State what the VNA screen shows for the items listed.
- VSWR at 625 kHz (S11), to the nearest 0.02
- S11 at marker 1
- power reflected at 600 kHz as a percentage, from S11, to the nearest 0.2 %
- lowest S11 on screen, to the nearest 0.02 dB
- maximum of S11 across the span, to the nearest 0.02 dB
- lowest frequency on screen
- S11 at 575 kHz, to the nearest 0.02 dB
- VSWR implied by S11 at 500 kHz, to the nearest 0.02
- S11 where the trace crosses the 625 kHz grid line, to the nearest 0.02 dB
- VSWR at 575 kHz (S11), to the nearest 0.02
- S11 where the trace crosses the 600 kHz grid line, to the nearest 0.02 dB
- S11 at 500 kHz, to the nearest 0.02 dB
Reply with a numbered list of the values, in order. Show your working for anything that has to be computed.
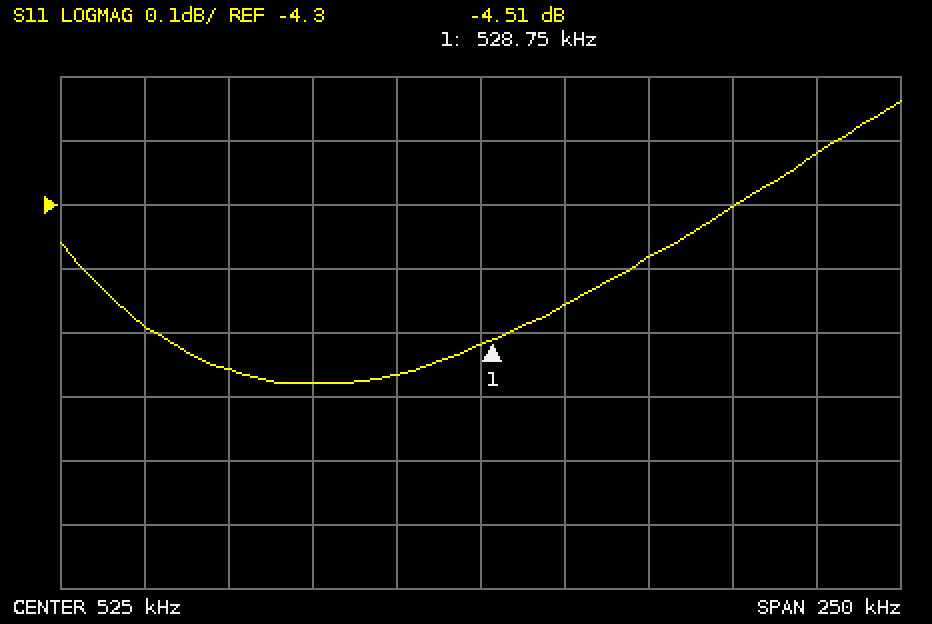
1. |Γ| = 10^(-4.22/20) = 0.6152; VSWR = (1 + 0.6152)/(1 − 0.6152) ≈ 4.20
2. -4.51 dB
3. 10^(-4.3/10) ≈ 37.2 %
4. -4.58 dB
5. -4.14 dB
6. 400 kHz
7. -4.38 dB
8. |Γ| = 10^(-4.56/20) = 0.5916; VSWR = (1 + 0.5916)/(1 − 0.5916) ≈ 3.90
9. -4.22 dB
10. |Γ| = 10^(-4.38/20) = 0.6039; VSWR = (1 + 0.6039)/(1 − 0.6039) ≈ 4.05, so 4.04 to the nearest 0.02
11. -4.30 dB
12. -4.56 dB
